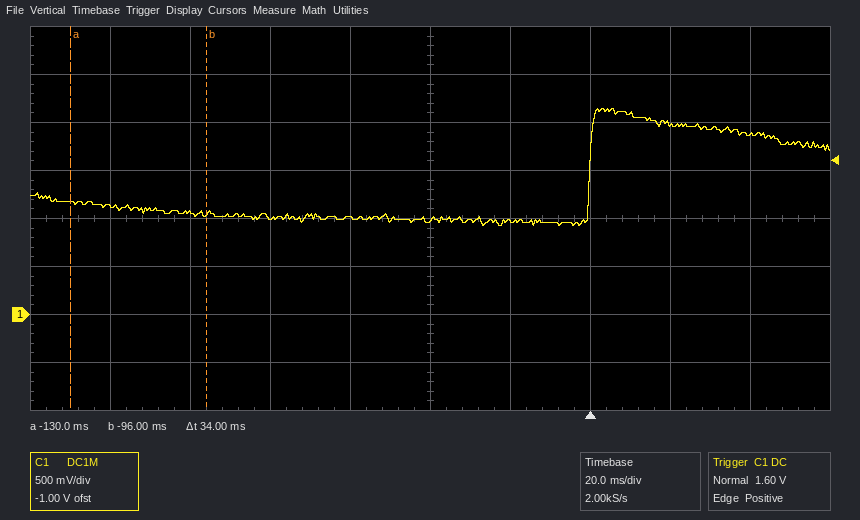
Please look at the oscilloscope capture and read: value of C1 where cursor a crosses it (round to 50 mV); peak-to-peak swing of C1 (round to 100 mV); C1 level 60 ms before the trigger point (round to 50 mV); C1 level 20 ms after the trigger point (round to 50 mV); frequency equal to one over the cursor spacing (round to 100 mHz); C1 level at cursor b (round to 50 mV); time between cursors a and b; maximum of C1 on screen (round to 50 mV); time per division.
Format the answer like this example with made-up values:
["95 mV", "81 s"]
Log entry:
["1.15 V", "1.20 V", "1.00 V", "2.00 V", "29.4 Hz", "1.05 V", "34 ms", "2.15 V", "20 ms"]
